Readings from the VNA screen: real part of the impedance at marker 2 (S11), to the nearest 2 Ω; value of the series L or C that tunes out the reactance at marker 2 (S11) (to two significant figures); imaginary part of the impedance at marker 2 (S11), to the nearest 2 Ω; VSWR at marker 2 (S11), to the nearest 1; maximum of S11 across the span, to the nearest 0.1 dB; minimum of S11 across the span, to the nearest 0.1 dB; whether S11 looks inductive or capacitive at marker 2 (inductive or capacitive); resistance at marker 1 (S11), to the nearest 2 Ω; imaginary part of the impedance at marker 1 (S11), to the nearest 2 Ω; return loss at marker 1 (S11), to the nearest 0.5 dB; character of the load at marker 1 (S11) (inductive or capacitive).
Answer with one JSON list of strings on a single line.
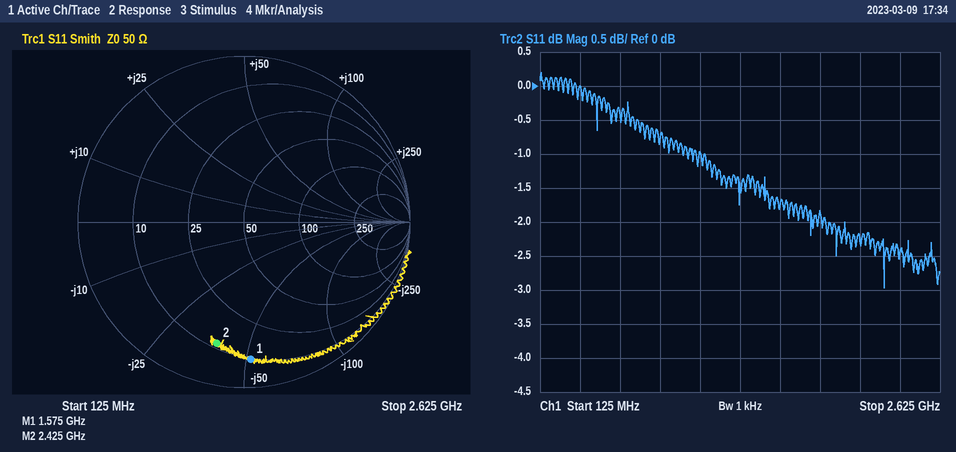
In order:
["12 Ω", "2.5 nH", "-38 Ω", "7", "0.2 dB", "-3.0 dB", "capacitive", "10 Ω", "-52 Ω", "1.5 dB", "capacitive"]
